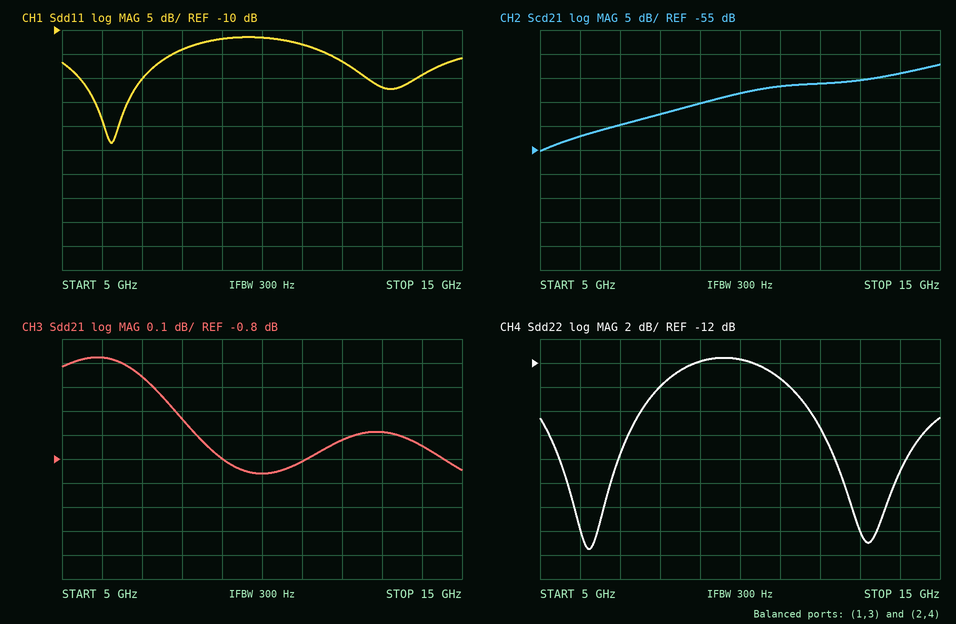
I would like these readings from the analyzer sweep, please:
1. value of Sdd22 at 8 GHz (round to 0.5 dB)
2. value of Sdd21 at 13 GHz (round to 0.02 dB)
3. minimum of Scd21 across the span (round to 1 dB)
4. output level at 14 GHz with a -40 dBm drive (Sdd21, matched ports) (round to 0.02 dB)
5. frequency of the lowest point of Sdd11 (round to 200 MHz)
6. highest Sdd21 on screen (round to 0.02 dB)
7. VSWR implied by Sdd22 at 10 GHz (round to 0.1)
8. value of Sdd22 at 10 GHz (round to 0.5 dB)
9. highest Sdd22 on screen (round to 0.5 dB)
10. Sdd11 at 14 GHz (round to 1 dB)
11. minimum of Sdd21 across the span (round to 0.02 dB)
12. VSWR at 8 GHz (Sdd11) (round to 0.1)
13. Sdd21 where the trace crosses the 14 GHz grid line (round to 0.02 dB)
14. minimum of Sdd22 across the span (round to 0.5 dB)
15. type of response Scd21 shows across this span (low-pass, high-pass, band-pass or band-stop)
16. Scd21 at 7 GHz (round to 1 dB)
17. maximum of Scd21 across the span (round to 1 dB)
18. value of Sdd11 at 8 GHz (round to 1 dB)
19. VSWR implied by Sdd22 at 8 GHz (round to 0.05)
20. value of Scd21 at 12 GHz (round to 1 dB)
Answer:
-14.0 dB
-0.68 dB
-55 dB
-40.74 dBm
6.2 GHz
-0.38 dB
1.7
-11.5 dB
-11.5 dB
-19 dB
-0.86 dB
1.5
-0.74 dB
-27.5 dB
high-pass
-50 dB
-37 dB
-14 dB
1.50
-41 dB
